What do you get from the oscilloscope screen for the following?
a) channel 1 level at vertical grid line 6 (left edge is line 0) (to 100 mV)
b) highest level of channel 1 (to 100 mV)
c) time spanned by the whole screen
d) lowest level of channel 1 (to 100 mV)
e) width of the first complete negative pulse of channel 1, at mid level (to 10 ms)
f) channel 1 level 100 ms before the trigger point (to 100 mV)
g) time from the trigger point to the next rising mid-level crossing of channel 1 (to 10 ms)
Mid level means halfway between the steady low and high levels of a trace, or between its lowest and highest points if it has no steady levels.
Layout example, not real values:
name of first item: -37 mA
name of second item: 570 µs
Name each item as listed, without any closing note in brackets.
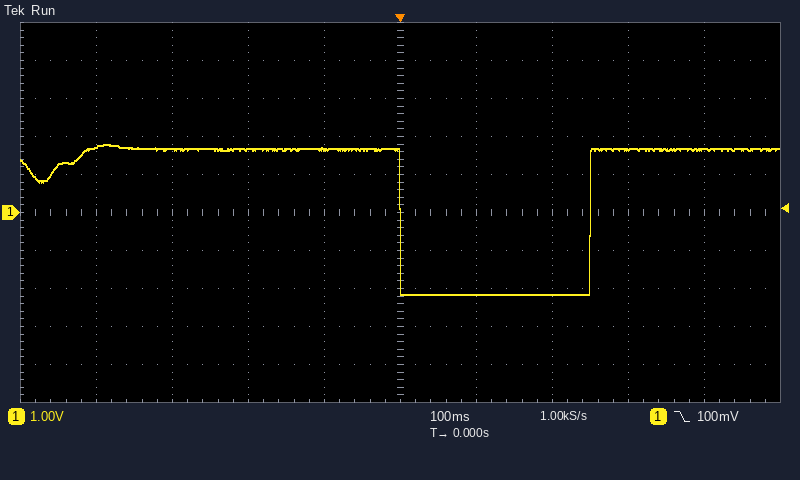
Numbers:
channel 1 level at vertical grid line 6 (left edge is line 0): -2.2 V
highest level of channel 1: 1.8 V
time spanned by the whole screen: 1 s
lowest level of channel 1: -2.2 V
width of the first complete negative pulse of channel 1, at mid level: 250 ms
channel 1 level 100 ms before the trigger point: 1.7 V
time from the trigger point to the next rising mid-level crossing of channel 1: 250 ms
